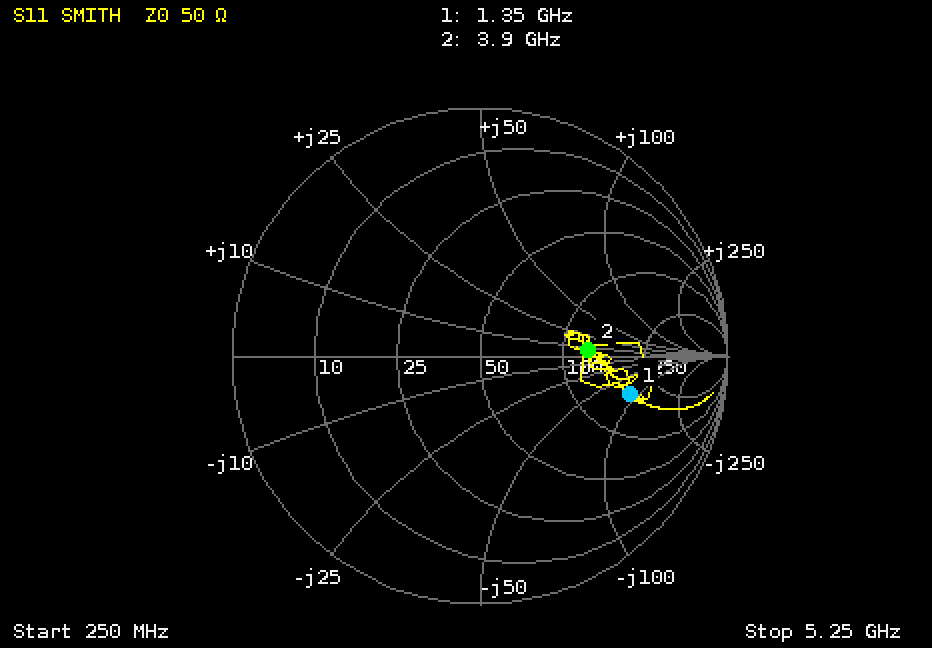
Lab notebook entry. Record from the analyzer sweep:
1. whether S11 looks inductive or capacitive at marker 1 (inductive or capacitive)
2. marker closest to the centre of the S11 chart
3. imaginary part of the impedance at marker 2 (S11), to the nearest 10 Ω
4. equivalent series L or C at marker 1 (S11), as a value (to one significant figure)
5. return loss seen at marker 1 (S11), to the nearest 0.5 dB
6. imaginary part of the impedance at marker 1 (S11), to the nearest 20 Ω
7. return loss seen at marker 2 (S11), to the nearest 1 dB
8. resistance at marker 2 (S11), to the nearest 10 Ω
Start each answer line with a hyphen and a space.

- capacitive
- marker 2
- +10 Ω
- 1 pF
- 4.0 dB
- -80 Ω
- 7 dB
- 130 Ω
